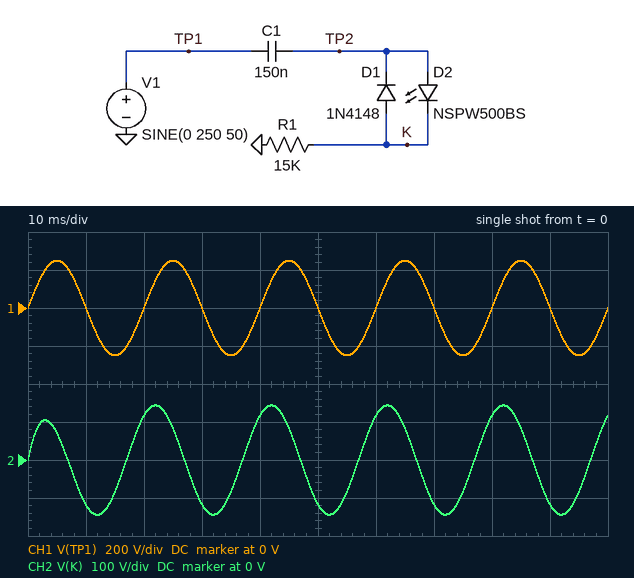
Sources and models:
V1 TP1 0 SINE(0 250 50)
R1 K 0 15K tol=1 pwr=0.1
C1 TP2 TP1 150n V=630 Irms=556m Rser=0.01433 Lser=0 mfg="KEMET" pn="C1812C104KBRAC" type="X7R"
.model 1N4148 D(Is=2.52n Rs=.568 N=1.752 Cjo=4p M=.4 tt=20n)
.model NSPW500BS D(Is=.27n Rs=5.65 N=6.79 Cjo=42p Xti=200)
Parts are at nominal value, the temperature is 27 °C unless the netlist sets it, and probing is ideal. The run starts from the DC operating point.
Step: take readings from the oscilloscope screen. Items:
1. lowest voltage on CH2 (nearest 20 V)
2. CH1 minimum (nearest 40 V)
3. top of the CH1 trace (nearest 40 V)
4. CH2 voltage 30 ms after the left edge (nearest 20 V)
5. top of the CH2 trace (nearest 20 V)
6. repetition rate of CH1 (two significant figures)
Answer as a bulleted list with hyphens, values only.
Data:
- -140 V
- -240 V
- 240 V
- -120 V
- 140 V
- 50 Hz
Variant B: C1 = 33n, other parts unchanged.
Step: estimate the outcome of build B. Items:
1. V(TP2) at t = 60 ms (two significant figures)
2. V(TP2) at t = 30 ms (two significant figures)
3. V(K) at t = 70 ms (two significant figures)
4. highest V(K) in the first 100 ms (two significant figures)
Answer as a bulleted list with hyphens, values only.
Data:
- 41 V
- -39 V
- -38 V
- 38 V
